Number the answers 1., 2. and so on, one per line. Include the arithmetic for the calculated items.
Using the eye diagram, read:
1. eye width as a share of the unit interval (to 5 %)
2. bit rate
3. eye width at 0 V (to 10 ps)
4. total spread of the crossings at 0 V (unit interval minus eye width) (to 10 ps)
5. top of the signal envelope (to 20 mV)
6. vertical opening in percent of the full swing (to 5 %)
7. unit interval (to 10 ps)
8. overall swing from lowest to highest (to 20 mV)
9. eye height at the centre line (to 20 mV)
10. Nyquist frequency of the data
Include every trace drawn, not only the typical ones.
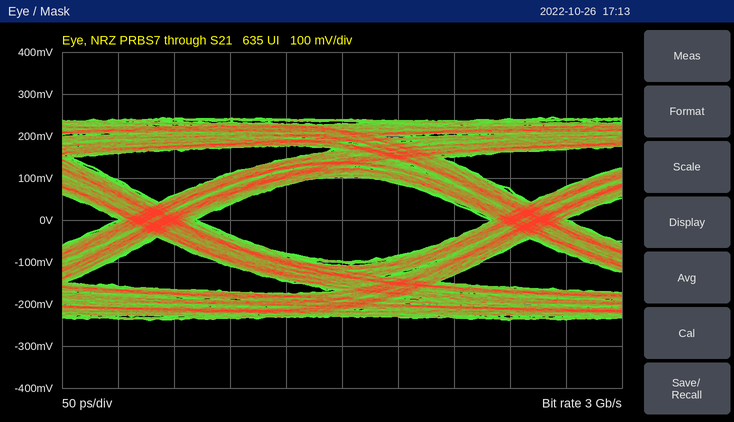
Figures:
1. 260 ps / 330 ps ≈ 78.8 %, so 80 % to the nearest 5 %
2. 3 Gb/s
3. 260 ps
4. 70 ps
5. 240 mV
6. 200 mV / 480 mV ≈ 41.7 %, so 40 % to the nearest 5 %
7. 330 ps
8. 480 mV
9. 200 mV
10. 1.5 GHz
